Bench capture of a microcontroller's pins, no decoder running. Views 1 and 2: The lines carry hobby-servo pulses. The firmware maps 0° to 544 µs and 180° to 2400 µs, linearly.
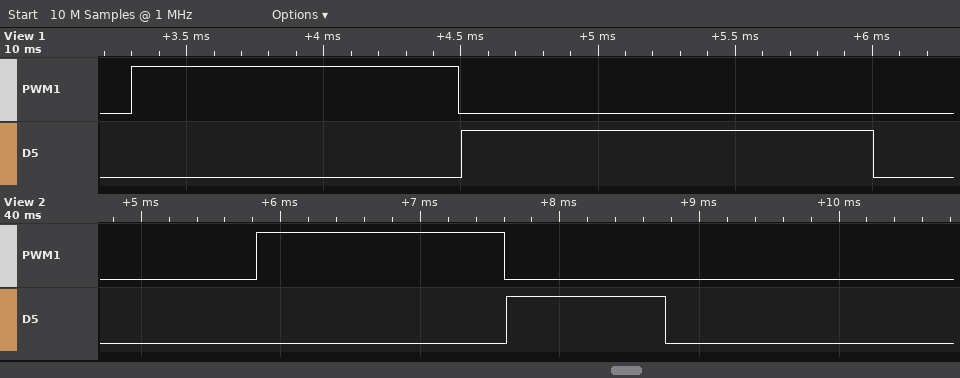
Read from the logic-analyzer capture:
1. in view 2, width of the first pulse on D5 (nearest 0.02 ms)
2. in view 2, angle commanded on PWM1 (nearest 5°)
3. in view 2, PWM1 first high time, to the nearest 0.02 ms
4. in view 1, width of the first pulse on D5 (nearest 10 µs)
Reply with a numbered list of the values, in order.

1. 1.14 ms
2. 120°
3. 1.78 ms
4. 1500 µs
